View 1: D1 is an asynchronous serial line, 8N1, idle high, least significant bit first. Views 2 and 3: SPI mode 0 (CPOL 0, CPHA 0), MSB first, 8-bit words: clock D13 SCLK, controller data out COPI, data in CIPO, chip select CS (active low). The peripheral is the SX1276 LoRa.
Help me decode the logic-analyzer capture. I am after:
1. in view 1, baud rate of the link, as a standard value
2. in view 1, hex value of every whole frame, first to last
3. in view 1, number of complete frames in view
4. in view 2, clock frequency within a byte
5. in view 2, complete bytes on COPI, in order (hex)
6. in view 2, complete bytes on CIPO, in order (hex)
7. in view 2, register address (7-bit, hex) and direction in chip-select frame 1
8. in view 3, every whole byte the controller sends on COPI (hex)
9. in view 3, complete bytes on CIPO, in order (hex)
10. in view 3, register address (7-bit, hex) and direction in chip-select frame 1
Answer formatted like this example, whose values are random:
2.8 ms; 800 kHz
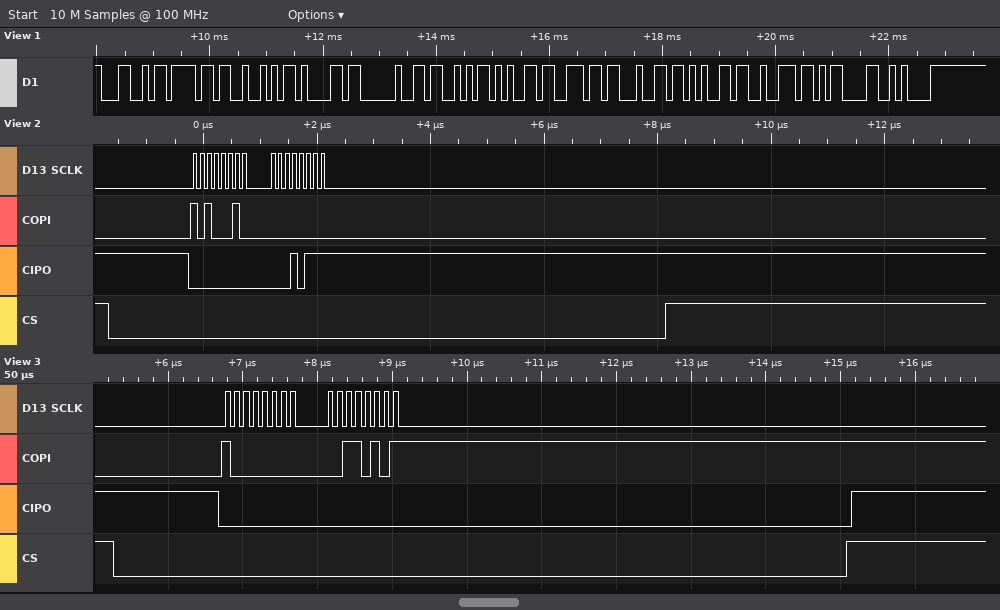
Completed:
9600 baud; 0x4C 0x6F 0x52 0x61 0x20 0x53 0x65 0x6E 0x64 0x65 0x72 0x0D 0x0A; 13; 8 MHz; A2 00; 00 17; 0x22 write; 80 35; 00 00; 0x00 write
